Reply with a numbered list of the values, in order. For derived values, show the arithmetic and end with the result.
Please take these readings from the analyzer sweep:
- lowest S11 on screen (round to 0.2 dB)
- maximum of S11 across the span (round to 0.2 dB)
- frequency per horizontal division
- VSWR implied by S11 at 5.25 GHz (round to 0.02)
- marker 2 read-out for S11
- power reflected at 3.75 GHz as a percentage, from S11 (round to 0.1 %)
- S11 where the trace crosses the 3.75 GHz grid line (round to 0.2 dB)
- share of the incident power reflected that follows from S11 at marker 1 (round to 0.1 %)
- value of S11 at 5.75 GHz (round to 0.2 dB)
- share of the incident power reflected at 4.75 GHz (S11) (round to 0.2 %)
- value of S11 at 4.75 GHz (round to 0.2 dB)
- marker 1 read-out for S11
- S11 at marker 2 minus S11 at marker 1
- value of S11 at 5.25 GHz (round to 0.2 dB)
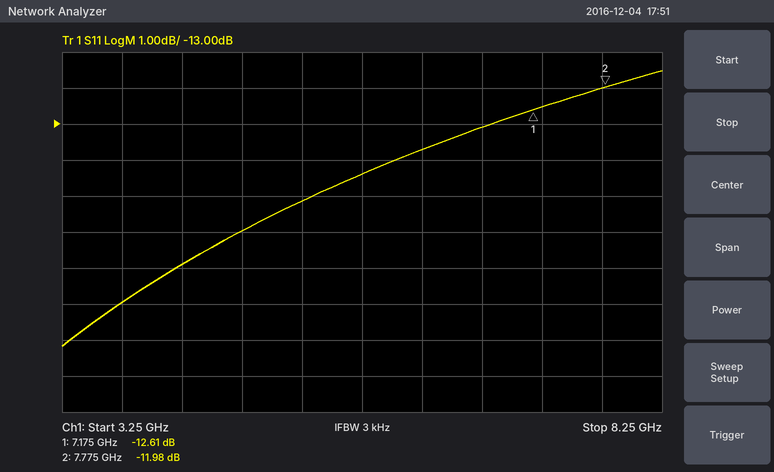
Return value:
1. -19.2 dB
2. -11.6 dB
3. 500 MHz
4. |Γ| = 10^(-15.2/20) = 0.1738; VSWR = (1 + 0.1738)/(1 − 0.1738) ≈ 1.42
5. -11.98 dB
6. 10^(-18/10) ≈ 1.6 %
7. -18.0 dB
8. 10^(-12.61/10) ≈ 5.5 %
9. -14.4 dB
10. 10^(-16/10) ≈ 2.51 %, so 2.6 % to the nearest 0.2 %
11. -16.0 dB
12. -12.61 dB
13. -11.98 − (-12.61) = 0.63 dB
14. -15.2 dB
